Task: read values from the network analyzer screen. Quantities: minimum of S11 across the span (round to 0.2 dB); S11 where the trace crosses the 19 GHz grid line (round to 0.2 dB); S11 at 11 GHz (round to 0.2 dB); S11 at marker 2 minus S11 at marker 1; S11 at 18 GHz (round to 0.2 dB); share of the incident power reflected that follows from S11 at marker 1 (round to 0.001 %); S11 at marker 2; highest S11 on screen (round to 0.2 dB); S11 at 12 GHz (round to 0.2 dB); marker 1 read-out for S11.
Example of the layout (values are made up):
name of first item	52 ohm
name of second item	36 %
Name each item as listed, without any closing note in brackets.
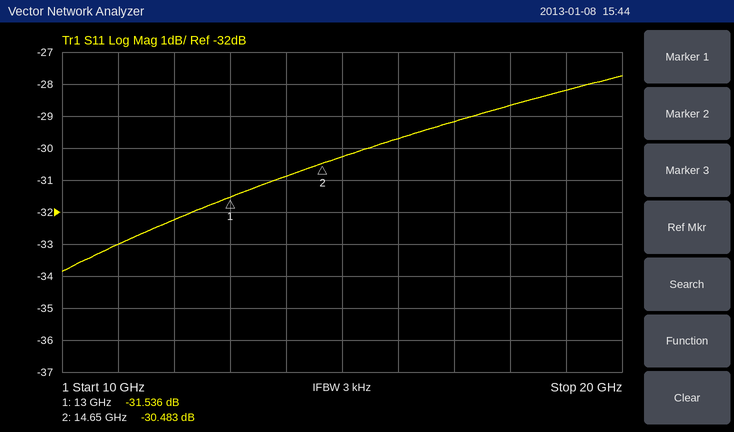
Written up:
minimum of S11 across the span	-33.8 dB
S11 where the trace crosses the 19 GHz grid line	-28.2 dB
S11 at 11 GHz	-33.0 dB
S11 at marker 2 minus S11 at marker 1	1.053 dB
S11 at 18 GHz	-28.6 dB
share of the incident power reflected that follows from S11 at marker 1	0.070 %
S11 at marker 2	-30.483 dB
highest S11 on screen	-27.8 dB
S11 at 12 GHz	-32.2 dB
marker 1 read-out for S11	-31.536 dB
